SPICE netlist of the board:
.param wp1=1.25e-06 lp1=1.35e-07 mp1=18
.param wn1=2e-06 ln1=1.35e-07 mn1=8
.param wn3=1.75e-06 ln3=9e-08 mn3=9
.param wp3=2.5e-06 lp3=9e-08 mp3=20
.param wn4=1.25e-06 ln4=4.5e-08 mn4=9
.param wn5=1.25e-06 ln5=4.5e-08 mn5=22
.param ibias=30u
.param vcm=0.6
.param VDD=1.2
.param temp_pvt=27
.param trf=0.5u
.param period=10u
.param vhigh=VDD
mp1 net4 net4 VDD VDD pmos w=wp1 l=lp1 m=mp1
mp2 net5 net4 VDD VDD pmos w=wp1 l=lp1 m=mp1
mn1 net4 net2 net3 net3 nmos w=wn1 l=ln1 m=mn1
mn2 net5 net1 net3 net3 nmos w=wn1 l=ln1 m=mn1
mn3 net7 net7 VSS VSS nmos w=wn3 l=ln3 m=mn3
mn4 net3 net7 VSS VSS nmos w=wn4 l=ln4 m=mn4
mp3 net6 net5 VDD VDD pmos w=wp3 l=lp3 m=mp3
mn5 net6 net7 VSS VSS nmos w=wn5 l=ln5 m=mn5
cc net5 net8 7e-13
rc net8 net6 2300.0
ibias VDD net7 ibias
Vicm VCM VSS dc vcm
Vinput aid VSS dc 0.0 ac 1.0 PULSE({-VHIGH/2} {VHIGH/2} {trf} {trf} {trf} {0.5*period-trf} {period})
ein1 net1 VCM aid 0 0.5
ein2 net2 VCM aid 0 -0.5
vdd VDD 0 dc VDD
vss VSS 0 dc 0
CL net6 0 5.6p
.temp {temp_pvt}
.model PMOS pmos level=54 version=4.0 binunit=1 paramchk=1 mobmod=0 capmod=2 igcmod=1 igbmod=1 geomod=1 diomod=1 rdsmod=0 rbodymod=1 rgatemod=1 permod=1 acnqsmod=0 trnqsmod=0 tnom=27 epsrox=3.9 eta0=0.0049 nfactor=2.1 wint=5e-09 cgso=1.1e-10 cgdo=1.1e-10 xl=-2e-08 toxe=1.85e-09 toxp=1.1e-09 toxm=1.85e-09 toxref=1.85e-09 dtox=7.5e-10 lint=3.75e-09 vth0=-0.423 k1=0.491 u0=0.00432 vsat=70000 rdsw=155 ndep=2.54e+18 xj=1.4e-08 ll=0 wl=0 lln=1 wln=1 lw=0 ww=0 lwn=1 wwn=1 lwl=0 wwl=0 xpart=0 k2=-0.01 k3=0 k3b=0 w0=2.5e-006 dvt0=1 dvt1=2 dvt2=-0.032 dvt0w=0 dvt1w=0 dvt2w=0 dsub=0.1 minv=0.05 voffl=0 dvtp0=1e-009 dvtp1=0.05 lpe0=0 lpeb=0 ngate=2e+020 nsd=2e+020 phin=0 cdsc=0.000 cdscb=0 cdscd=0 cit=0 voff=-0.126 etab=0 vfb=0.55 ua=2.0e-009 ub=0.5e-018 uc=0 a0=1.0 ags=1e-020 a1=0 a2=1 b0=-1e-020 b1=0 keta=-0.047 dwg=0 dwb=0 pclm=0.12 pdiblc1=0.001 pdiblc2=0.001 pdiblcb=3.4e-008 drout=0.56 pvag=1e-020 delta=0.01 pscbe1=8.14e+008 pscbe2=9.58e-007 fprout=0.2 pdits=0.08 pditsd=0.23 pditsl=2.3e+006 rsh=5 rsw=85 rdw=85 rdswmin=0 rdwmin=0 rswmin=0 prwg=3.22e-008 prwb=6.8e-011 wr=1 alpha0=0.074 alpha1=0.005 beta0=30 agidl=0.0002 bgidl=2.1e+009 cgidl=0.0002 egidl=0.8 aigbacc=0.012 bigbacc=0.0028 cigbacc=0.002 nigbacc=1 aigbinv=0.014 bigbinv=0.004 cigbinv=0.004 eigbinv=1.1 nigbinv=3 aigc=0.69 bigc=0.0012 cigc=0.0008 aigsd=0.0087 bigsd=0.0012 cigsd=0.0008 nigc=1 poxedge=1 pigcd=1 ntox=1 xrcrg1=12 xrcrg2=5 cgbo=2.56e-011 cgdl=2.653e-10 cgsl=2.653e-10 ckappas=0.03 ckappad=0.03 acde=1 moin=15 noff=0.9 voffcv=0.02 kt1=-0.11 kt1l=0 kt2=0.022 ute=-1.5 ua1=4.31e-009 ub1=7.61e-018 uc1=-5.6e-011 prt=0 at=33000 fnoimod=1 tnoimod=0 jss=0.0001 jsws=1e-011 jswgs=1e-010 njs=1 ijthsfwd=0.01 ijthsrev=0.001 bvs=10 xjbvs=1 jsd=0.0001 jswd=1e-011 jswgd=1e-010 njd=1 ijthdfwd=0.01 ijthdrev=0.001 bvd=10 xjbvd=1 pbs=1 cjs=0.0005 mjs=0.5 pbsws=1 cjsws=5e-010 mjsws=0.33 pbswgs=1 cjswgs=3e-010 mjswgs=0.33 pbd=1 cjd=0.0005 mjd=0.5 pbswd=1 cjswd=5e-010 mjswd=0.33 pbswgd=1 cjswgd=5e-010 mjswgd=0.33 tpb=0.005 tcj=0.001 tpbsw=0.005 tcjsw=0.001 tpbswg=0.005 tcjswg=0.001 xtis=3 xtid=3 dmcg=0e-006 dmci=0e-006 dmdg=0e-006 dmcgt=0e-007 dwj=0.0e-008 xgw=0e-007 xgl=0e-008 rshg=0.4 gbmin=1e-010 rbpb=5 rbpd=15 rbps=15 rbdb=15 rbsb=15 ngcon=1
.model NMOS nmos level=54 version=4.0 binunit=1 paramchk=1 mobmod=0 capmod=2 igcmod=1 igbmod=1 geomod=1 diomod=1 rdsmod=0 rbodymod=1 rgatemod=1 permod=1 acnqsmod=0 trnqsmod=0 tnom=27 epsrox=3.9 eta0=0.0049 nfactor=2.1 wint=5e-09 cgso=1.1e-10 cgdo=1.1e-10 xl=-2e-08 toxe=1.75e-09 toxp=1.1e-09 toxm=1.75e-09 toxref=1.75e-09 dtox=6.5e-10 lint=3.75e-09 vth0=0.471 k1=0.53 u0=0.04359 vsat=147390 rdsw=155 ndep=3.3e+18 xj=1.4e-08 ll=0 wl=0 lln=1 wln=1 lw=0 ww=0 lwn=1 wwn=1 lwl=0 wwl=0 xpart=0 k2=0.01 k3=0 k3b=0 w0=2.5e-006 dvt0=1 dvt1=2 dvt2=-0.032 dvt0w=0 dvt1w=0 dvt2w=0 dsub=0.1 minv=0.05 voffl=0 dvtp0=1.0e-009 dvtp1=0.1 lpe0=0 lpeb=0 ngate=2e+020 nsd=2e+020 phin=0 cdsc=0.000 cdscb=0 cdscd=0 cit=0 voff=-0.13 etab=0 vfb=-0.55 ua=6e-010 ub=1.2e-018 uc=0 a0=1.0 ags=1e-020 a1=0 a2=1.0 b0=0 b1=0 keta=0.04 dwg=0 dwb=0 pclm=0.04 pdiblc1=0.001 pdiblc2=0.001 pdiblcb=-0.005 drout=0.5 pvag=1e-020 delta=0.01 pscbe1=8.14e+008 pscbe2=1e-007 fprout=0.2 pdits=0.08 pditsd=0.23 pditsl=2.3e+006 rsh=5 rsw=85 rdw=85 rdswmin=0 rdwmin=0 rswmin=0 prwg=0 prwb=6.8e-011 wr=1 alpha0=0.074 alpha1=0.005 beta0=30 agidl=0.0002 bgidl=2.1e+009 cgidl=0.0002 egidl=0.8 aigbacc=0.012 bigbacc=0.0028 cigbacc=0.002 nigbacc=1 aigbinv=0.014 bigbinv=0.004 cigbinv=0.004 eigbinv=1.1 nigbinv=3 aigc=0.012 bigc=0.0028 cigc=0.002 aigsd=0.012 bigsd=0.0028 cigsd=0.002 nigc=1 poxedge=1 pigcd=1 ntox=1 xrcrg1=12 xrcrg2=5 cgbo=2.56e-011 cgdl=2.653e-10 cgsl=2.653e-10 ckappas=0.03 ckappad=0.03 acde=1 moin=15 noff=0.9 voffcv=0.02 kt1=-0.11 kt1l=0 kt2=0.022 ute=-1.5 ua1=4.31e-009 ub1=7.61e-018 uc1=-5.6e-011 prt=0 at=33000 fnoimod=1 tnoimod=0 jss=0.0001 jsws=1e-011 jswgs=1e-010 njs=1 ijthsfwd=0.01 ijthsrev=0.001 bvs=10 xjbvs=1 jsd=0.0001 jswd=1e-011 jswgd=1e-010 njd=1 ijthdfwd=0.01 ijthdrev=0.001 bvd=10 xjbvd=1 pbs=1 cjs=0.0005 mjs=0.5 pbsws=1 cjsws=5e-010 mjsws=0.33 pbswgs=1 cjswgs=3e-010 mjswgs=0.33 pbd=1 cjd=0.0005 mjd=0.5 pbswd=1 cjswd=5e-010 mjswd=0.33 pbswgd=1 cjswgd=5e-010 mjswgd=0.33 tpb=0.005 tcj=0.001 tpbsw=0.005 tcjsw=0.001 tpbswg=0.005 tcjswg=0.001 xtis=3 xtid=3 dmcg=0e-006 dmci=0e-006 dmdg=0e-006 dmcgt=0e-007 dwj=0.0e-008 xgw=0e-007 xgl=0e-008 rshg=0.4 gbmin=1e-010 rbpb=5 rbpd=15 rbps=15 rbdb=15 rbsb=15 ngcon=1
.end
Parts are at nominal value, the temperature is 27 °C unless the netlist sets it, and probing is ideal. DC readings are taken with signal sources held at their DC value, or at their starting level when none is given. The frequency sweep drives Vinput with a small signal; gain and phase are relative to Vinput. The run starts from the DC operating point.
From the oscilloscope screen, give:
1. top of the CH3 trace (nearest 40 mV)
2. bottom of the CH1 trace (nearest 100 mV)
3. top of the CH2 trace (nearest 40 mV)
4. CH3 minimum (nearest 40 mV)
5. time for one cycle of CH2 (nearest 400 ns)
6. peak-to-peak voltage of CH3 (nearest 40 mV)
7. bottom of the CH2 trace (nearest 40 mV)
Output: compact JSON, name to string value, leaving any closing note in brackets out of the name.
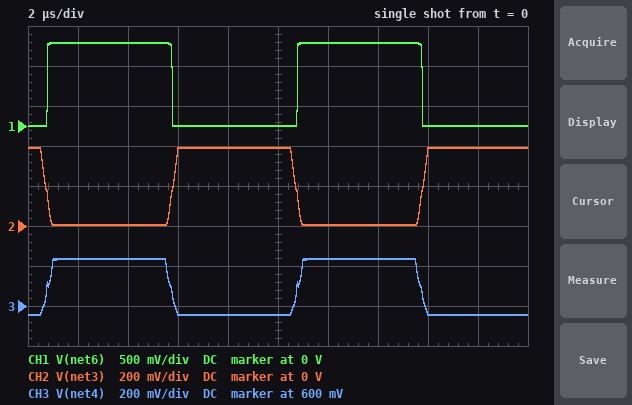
{"top of the CH3 trace": "840 mV", "bottom of the CH1 trace": "0 V", "top of the CH2 trace": "400 mV", "CH3 minimum": "560 mV", "time for one cycle of CH2": "10.0 µs", "peak-to-peak voltage of CH3": "280 mV", "bottom of the CH2 trace": "0 V"}
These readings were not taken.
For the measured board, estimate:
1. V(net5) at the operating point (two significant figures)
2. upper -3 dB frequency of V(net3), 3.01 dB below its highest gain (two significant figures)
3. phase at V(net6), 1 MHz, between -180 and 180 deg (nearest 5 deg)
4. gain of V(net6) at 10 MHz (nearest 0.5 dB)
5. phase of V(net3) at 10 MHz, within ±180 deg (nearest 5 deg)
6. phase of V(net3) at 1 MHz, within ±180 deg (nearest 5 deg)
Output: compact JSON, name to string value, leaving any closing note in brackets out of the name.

{"V(net5) at the operating point": "690 mV", "upper -3 dB frequency of V(net3), 3.01 dB below its highest gain": "800 kHz", "phase at V(net6), 1 MHz, between -180 and 180 deg": "-50 deg", "gain of V(net6) at 10 MHz": "25.0 dB", "phase of V(net3) at 10 MHz, within ±180 deg": "150 deg", "phase of V(net3) at 1 MHz, within ±180 deg": "135 deg"}
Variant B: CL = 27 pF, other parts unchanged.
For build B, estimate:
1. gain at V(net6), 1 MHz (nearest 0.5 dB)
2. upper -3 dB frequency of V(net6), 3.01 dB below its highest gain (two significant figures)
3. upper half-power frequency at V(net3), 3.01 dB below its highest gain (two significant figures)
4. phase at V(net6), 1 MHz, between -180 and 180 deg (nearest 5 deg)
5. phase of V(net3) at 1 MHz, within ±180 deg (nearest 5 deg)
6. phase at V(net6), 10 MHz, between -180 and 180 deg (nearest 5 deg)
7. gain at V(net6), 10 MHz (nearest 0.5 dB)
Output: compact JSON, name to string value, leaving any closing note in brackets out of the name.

{"gain at V(net6), 1 MHz": "42.5 dB", "upper -3 dB frequency of V(net6), 3.01 dB below its highest gain": "730 kHz", "upper half-power frequency at V(net3), 3.01 dB below its highest gain": "760 kHz", "phase at V(net6), 1 MHz, between -180 and 180 deg": "-55 deg", "phase of V(net3) at 1 MHz, within ±180 deg": "140 deg", "phase at V(net6), 10 MHz, between -180 and 180 deg": "-100 deg", "gain at V(net6), 10 MHz": "24.0 dB"}
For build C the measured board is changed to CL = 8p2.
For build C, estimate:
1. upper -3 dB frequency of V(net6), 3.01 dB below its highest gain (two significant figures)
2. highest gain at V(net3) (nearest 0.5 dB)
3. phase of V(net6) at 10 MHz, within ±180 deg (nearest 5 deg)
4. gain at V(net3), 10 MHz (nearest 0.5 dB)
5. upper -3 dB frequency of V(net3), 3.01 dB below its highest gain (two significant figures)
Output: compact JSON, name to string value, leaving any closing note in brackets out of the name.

{"upper -3 dB frequency of V(net6), 3.01 dB below its highest gain": "780 kHz", "highest gain at V(net3)": "-13.5 dB", "phase of V(net6) at 10 MHz, within ±180 deg": "-90 deg", "gain at V(net3), 10 MHz": "-30.0 dB", "upper -3 dB frequency of V(net3), 3.01 dB below its highest gain": "790 kHz"}
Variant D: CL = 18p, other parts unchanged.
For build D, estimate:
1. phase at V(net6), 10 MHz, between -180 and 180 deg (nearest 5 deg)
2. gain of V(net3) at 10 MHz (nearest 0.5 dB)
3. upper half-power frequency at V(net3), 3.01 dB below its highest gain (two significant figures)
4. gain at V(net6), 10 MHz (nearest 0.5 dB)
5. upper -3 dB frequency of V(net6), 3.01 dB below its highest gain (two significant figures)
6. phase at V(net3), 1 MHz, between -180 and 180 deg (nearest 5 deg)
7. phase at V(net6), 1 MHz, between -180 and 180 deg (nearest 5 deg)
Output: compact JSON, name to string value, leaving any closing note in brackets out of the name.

{"phase at V(net6), 10 MHz, between -180 and 180 deg": "-95 deg", "gain of V(net3) at 10 MHz": "-28.5 dB", "upper half-power frequency at V(net3), 3.01 dB below its highest gain": "770 kHz", "gain at V(net6), 10 MHz": "24.5 dB", "upper -3 dB frequency of V(net6), 3.01 dB below its highest gain": "750 kHz", "phase at V(net3), 1 MHz, between -180 and 180 deg": "140 deg", "phase at V(net6), 1 MHz, between -180 and 180 deg": "-55 deg"}
